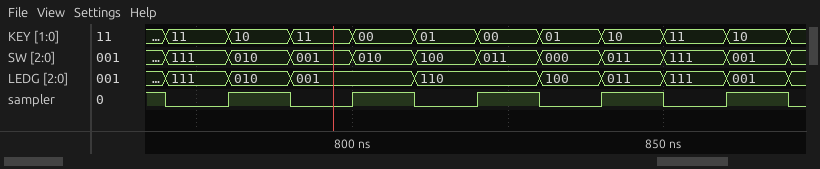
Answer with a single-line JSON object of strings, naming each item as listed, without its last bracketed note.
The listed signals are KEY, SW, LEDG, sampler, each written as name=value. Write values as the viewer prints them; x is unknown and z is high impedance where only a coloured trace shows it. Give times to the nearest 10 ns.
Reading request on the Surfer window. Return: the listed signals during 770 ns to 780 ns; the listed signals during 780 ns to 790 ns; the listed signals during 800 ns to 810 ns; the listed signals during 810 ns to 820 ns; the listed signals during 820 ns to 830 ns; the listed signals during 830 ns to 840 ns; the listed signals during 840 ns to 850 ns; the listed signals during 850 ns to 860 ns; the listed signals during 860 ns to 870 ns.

{"the listed signals during 770 ns to 780 ns": "KEY=11, SW=111, LEDG=111, sampler=0", "the listed signals during 780 ns to 790 ns": "KEY=10, SW=010, LEDG=010, sampler=1", "the listed signals during 800 ns to 810 ns": "KEY=00, SW=010, LEDG=001, sampler=1", "the listed signals during 810 ns to 820 ns": "KEY=01, SW=100, LEDG=110, sampler=0", "the listed signals during 820 ns to 830 ns": "KEY=00, SW=011, LEDG=110, sampler=1", "the listed signals during 830 ns to 840 ns": "KEY=01, SW=000, LEDG=100, sampler=0", "the listed signals during 840 ns to 850 ns": "KEY=10, SW=011, LEDG=011, sampler=1", "the listed signals during 850 ns to 860 ns": "KEY=11, SW=111, LEDG=111, sampler=0", "the listed signals during 860 ns to 870 ns": "KEY=10, SW=001, LEDG=001, sampler=1"}
